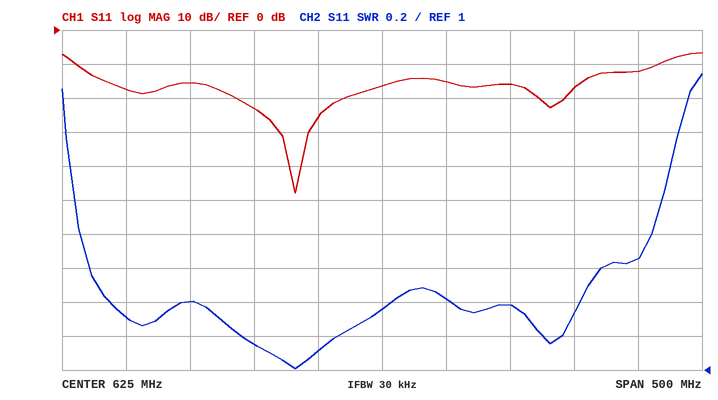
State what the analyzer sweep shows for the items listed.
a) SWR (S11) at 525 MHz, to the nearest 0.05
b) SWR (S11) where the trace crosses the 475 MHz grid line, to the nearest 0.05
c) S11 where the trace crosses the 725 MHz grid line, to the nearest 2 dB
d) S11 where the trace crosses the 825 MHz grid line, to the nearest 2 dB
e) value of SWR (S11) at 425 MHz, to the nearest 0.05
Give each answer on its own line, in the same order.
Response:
1.15
1.40
-16 dB
-12 dB
1.30
